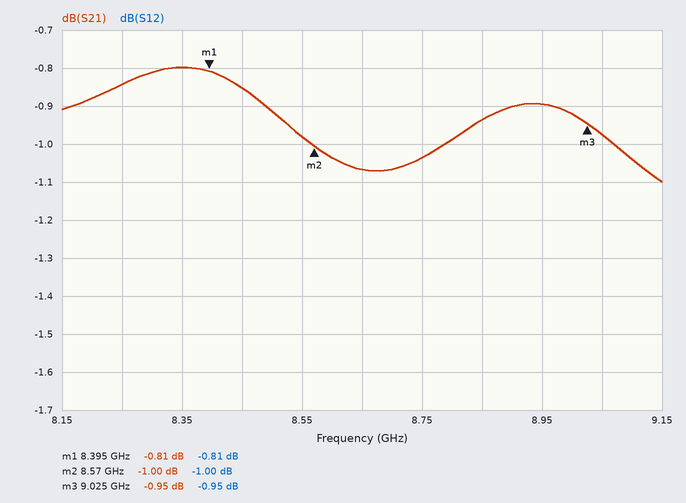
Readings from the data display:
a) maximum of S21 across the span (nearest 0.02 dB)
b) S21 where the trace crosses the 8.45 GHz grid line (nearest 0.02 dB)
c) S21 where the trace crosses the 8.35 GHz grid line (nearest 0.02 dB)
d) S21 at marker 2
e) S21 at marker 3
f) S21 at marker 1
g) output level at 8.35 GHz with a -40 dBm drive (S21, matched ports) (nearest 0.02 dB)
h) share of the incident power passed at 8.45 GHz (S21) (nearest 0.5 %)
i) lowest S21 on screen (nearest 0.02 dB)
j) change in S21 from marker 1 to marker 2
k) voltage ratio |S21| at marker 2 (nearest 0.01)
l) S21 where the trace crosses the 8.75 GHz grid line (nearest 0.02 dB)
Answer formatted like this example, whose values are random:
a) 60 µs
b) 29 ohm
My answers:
a) -0.80 dB
b) -0.86 dB
c) -0.80 dB
d) -1.00 dB
e) -0.95 dB
f) -0.81 dB
g) -40.80 dBm
h) 82.0 %
i) -1.10 dB
j) -0.19 dB
k) 0.89
l) -1.04 dB
